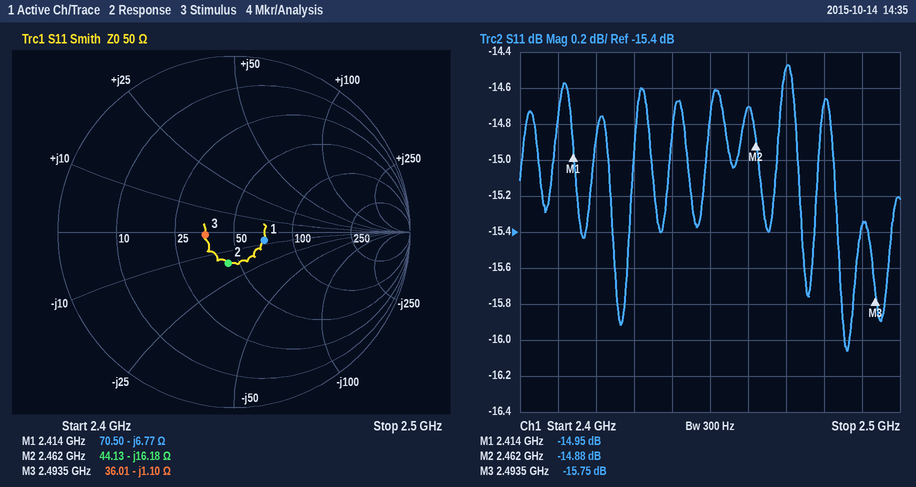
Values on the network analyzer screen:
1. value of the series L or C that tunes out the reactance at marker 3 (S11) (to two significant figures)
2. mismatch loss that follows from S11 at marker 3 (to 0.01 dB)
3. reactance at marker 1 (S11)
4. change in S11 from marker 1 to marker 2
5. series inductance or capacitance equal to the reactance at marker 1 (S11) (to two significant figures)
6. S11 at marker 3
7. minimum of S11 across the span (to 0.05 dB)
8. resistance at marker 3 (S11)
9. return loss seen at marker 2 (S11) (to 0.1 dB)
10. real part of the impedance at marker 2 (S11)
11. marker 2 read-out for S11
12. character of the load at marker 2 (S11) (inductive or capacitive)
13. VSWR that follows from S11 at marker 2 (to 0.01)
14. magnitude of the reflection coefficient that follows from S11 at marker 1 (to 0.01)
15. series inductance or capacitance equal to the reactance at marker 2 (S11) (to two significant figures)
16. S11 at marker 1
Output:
70 pH
0.12 dB
-6.77 Ω
0.07 dB
9.7 pF
-15.75 dB
-16.05 dB
36.01 Ω
14.9 dB
44.13 Ω
-14.88 dB
capacitive
1.44
0.18
4.0 pF
-14.95 dB
